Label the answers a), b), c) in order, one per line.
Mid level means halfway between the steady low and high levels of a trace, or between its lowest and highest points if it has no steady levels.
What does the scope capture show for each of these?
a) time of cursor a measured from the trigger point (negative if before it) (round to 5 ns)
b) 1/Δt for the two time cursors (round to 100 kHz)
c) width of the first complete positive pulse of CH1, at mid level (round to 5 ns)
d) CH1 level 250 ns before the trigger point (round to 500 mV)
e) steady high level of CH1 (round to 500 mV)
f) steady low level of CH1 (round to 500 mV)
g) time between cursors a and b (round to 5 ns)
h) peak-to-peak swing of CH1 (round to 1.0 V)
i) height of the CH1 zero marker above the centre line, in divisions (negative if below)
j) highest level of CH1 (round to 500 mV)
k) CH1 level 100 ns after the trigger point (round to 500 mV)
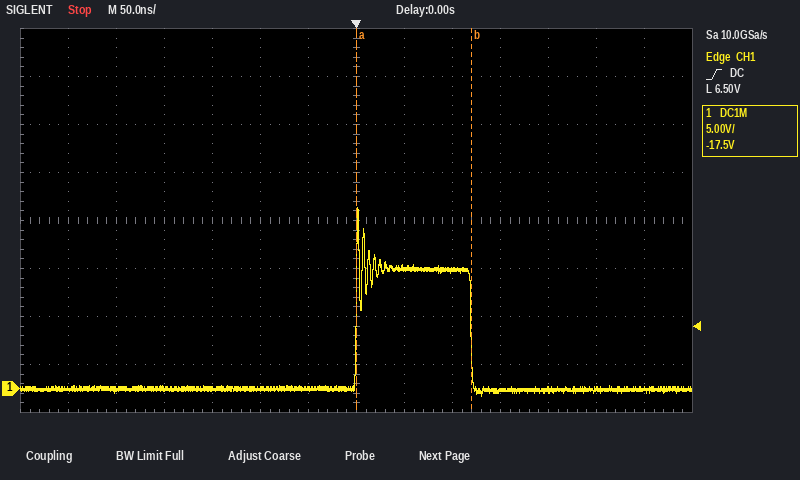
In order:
a) 0 ns
b) 8.3 MHz
c) 120 ns
d) 0.0 V
e) 12.5 V
f) 0.0 V
g) 120 ns
h) 20.0 V
i) -3.5 div
j) 19.0 V
k) 12.5 V
